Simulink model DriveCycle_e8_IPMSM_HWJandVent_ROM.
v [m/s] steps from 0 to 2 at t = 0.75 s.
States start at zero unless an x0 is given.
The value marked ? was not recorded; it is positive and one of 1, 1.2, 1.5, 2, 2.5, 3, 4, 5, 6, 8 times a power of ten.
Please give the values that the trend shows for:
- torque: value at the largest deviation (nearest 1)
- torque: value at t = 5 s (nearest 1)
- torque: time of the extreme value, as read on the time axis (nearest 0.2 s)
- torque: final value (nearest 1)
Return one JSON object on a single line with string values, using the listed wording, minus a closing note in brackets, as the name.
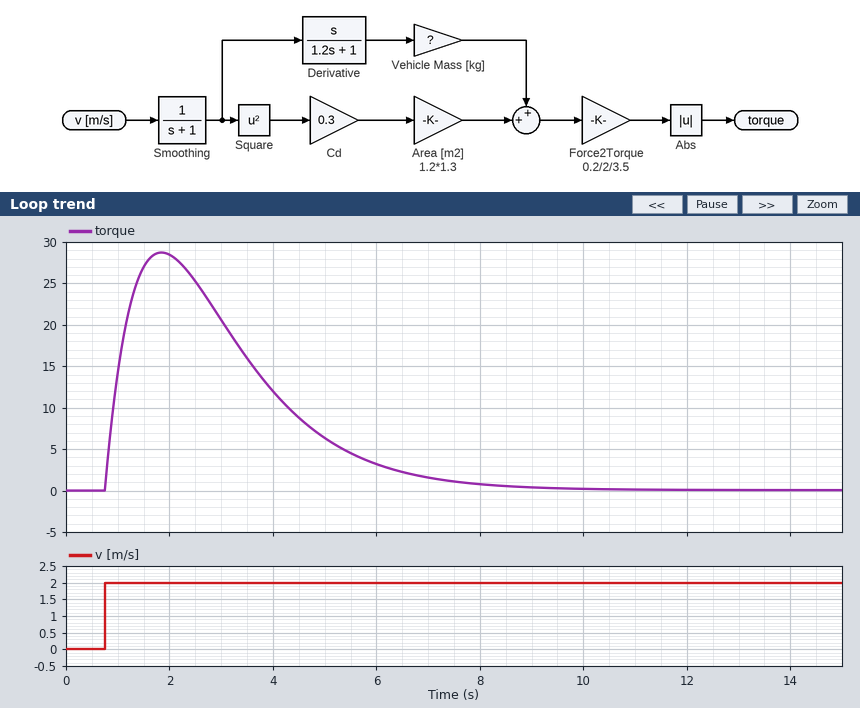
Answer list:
{"torque: value at the largest deviation": "29", "torque: value at t = 5 s": "6", "torque: time of the extreme value, as read on the time axis": "1.8 s", "torque: final value": "0"}
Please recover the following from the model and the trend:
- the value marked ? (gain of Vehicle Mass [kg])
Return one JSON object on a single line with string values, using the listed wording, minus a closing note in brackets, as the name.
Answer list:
{"the value marked ?": "1500"}
